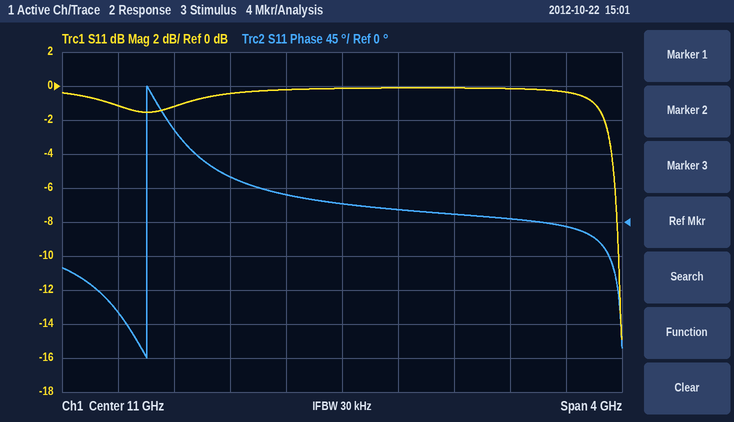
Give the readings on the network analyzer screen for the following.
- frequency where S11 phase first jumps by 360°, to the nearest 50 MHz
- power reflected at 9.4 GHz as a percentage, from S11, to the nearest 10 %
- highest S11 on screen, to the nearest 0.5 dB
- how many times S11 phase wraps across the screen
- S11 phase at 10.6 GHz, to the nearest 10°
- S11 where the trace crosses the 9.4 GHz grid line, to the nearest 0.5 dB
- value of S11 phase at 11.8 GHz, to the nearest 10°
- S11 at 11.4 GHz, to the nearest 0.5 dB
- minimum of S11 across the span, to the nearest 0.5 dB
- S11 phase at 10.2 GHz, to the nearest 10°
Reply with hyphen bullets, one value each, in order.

- 9.60 GHz
- 80 %
- 0.0 dB
- 1
- 40°
- -1.0 dB
- 10°
- 0.0 dB
- -15.0 dB
- 60°
